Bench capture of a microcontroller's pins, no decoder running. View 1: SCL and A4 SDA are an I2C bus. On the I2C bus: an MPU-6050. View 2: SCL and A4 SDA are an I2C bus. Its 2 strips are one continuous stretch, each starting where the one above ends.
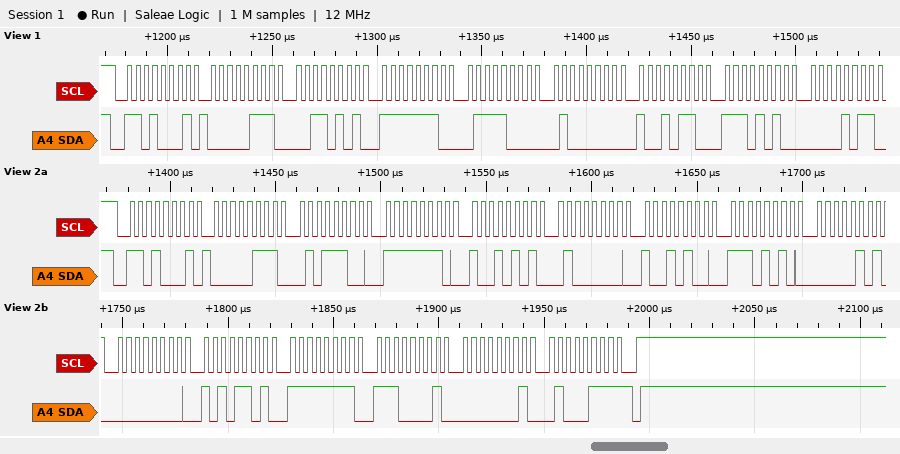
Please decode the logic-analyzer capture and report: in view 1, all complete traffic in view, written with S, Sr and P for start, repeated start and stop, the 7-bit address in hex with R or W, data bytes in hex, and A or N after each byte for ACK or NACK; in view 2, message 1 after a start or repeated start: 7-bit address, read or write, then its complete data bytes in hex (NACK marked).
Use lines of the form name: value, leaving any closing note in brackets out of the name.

in view 1, all complete traffic in view, written with S, Sr and P for start, repeated start and stop, the 7-bit address in hex with R or W, data bytes in hex, and A or N after each byte for ACK or NACK: S 68R A 07 A 35 A FE A 78 A 40 A 96 A EA A 0B A
in view 2, message 1 after a start or repeated start: 7-bit address, read or write, then its complete data bytes in hex: 0x68 read: 07 5C FE 95 40 94 EA 05 00 AD FF E1 01 47 NACK
